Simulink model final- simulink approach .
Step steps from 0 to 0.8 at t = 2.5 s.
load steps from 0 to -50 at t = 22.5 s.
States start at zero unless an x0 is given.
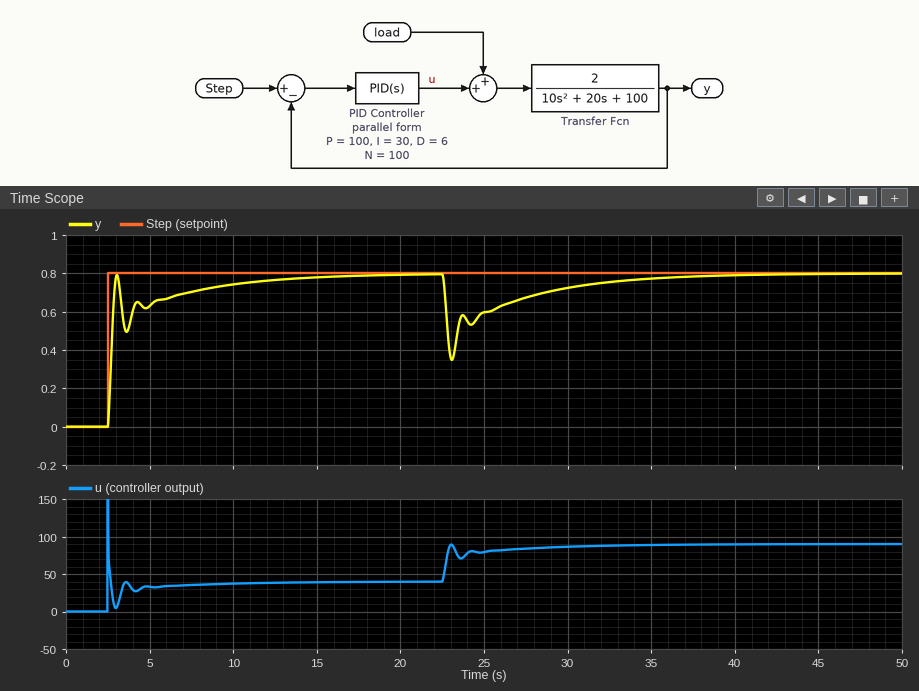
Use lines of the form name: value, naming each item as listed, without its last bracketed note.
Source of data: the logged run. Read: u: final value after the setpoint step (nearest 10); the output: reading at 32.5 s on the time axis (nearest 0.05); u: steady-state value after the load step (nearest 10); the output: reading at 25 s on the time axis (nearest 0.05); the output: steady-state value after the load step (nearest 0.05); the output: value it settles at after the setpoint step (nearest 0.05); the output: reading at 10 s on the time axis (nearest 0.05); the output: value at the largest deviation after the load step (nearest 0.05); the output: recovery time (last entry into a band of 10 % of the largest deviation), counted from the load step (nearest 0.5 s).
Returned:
u: final value after the setpoint step: 40
the output: reading at 32.5 s on the time axis: 0.75
u: steady-state value after the load step: 90
the output: reading at 25 s on the time axis: 0.60
the output: steady-state value after the load step: 0.80
the output: value it settles at after the setpoint step: 0.80
the output: reading at 10 s on the time axis: 0.75
the output: value at the largest deviation after the load step: 0.35
the output: recovery time (last entry into a band of 10 % of the largest deviation), counted from the load step: 10.0 s
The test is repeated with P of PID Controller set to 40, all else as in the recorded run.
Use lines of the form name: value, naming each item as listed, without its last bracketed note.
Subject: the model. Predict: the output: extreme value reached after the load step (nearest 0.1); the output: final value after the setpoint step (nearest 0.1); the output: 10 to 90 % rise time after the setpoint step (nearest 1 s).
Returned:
the output: extreme value reached after the load step: 0.1
the output: final value after the setpoint step: 0.8
the output: 10 to 90 % rise time after the setpoint step: 5 s
